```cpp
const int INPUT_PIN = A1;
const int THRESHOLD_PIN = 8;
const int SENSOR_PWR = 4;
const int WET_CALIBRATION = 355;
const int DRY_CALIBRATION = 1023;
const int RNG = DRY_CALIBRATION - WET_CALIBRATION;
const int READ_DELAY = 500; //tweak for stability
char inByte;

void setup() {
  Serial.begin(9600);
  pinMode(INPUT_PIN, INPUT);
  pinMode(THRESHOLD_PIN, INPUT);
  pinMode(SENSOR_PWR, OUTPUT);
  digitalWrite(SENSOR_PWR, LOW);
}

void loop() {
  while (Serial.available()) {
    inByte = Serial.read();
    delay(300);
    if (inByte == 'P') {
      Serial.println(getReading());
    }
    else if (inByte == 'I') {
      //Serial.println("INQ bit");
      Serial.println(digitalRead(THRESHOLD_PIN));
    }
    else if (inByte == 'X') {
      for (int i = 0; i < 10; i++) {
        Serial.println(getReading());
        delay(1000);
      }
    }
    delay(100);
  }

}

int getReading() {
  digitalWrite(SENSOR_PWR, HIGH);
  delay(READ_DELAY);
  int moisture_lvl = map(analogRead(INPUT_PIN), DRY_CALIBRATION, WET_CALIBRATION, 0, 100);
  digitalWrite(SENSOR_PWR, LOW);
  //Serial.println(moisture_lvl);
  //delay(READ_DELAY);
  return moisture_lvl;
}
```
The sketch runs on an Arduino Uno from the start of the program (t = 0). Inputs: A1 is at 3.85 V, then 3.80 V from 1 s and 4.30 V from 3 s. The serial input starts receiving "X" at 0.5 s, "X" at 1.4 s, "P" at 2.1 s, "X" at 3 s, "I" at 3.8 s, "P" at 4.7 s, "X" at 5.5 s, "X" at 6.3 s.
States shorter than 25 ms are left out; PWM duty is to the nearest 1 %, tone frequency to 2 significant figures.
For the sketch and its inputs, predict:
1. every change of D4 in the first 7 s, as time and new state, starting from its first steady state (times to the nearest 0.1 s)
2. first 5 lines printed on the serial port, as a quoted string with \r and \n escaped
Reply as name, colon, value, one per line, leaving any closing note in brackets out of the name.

every change of D4 in the first 7 s, as time and new state, starting from its first steady state: 0 s low; 0.8 s high; 1.3 s low; 2.3 s high; 2.8 s low; 3.8 s high; 4.3 s low; 5.3 s high; 5.8 s low; 6.8 s high
first 5 lines printed on the serial port, as a quoted string with \r and \n escaped: "36\r\n36\r\n21\r\n21\r\n21\r\n"
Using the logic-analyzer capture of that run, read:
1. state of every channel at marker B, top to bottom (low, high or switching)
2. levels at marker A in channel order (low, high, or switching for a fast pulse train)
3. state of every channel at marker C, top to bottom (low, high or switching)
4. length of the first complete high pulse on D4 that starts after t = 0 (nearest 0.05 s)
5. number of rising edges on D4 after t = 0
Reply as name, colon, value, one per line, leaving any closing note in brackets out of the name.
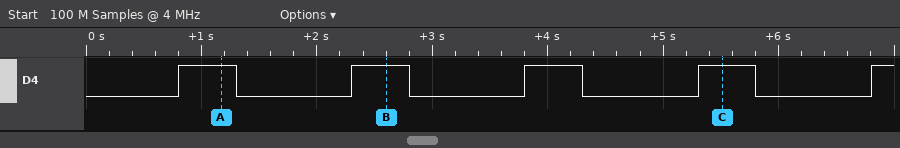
state of every channel at marker B, top to bottom: D4 high
levels at marker A in channel order: D4 high
state of every channel at marker C, top to bottom: D4 high
length of the first complete high pulse on D4 that starts after t = 0: 0.50 s
number of rising edges on D4 after t = 0: 5
